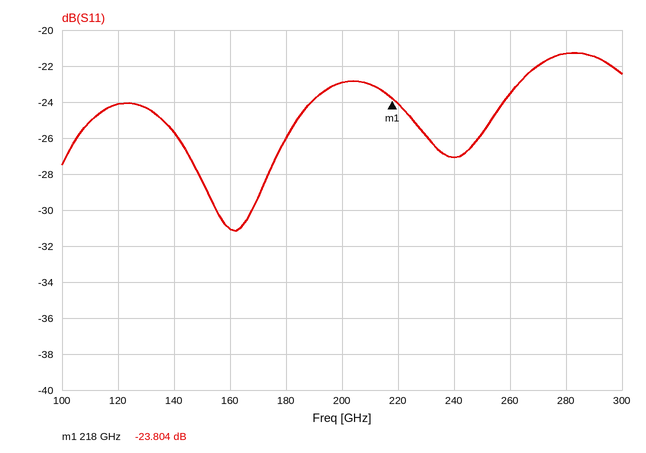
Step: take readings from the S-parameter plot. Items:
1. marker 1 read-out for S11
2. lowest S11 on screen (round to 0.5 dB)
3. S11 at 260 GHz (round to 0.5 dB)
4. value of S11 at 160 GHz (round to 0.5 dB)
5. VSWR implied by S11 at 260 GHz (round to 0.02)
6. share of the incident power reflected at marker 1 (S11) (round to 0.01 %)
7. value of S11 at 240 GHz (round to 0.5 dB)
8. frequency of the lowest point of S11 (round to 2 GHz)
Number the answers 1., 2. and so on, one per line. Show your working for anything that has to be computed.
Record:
1. -23.804 dB
2. -31.0 dB
3. -23.5 dB
4. -31.0 dB
5. |Γ| = 10^(-23.5/20) = 0.0668; VSWR = (1 + 0.0668)/(1 − 0.0668) ≈ 1.14
6. 10^(-23.804/10) ≈ 0.42 %
7. -27.0 dB
8. 162 GHz
